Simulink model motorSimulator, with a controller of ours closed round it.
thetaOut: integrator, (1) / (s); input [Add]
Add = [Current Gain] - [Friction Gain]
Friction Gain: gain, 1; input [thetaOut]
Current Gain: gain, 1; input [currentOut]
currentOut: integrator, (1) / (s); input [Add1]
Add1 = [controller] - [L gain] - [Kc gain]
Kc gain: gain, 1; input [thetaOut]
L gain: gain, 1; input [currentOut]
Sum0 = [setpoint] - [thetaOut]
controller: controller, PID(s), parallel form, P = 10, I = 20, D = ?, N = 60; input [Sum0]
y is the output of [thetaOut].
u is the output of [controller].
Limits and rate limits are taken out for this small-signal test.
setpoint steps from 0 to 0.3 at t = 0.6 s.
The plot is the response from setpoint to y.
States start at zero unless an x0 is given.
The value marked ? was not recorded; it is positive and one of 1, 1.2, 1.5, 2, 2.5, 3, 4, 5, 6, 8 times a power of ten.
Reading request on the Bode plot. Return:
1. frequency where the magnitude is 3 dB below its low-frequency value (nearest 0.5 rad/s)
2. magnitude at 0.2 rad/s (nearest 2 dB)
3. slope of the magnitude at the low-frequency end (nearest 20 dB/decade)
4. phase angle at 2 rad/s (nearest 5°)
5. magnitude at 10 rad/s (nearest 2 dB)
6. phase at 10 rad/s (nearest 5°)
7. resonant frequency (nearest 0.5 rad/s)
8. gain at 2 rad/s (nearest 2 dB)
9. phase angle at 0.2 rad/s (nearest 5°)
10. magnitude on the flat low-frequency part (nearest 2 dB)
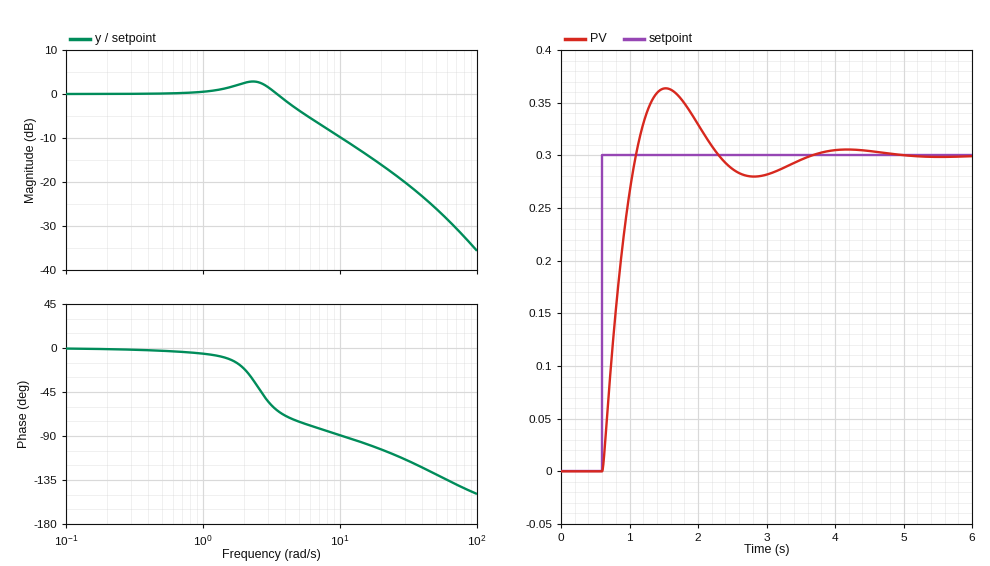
4.5 rad/s
0 dB
0 dB/decade
-20°
-10 dB
-90°
2.5 rad/s
2 dB
0°
0 dB
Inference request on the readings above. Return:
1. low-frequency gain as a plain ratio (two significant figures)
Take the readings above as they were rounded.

1.0
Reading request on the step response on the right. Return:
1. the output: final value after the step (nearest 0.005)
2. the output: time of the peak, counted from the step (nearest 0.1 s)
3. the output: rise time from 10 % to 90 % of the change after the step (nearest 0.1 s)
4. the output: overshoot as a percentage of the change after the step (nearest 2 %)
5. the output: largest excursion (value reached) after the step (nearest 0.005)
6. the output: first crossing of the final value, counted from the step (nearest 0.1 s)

0.300
0.9 s
0.4 s
22 %
0.365
0.5 s
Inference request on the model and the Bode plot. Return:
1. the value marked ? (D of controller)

3
